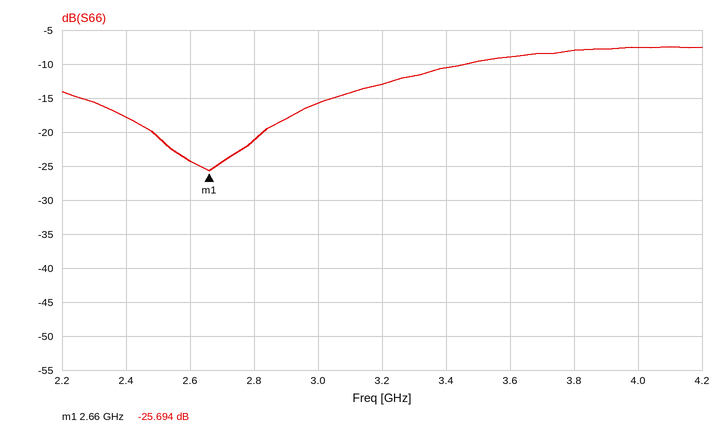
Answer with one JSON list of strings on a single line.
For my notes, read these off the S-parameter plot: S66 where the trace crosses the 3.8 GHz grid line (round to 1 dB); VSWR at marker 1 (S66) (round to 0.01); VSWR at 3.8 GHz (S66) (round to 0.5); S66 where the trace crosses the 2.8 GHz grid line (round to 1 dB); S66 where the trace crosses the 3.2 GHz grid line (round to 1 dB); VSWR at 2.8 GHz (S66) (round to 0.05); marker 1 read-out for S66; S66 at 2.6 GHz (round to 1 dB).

["-8 dB", "1.11", "2.5", "-21 dB", "-13 dB", "1.20", "-25.694 dB", "-24 dB"]
